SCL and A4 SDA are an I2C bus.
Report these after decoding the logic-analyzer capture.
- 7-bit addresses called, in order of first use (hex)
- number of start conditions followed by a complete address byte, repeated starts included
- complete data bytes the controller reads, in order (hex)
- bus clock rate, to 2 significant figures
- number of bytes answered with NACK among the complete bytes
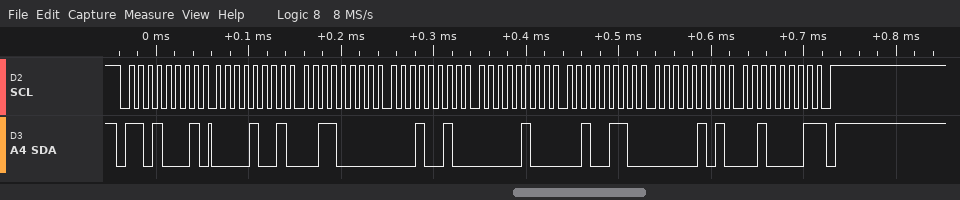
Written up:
0x68
1
09 30 12 04 26 05 21
100 kHz
1
